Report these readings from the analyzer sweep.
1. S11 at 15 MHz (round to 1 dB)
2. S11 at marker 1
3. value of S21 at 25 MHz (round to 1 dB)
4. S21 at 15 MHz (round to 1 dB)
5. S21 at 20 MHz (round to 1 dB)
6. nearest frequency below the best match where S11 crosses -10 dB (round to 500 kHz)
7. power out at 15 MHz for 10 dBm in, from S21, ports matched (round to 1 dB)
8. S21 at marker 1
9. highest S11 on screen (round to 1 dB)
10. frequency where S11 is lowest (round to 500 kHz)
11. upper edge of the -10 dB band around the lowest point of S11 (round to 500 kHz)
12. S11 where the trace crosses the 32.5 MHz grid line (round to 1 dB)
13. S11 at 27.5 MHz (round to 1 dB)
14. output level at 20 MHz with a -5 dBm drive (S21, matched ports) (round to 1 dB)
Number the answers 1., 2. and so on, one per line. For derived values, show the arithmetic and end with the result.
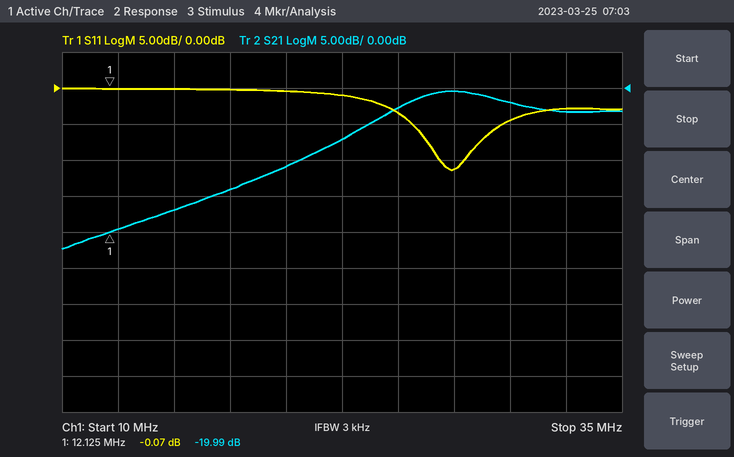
1. 0 dB
2. -0.07 dB
3. -3 dB
4. -17 dB
5. -11 dB
6. 27.0 MHz
7. 10 dBm + (-17 dB) = -7 dBm
8. -19.99 dB
9. 0 dB
10. 27.5 MHz
11. 28.0 MHz
12. -3 dB
13. -11 dB
14. -5 dBm + (-11 dB) = -16 dBm
